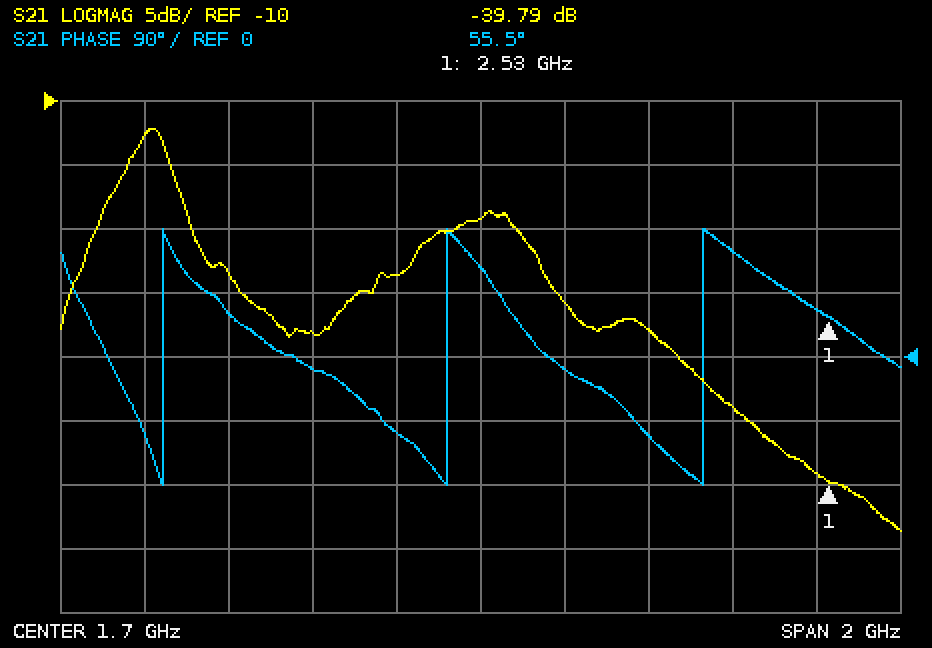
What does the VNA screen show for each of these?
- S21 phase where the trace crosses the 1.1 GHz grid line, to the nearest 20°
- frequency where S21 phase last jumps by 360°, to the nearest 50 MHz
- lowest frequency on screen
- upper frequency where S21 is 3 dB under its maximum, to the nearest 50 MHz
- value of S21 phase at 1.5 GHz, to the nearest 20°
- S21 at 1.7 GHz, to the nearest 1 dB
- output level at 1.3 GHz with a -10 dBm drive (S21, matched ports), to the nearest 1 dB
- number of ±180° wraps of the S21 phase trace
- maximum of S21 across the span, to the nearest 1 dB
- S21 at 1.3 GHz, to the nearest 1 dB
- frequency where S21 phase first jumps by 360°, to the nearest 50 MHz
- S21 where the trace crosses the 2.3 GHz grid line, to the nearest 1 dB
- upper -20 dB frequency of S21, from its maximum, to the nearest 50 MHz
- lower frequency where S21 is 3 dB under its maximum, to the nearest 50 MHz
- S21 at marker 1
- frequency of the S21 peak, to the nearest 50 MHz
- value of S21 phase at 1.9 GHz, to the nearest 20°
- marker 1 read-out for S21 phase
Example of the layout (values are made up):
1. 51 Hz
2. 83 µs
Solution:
1. 60°
2. 2.25 GHz
3. 700 MHz
4. 950 MHz
5. -100°
6. -19 dB
7. -38 dBm
8. 3
9. -12 dB
10. -28 dB
11. 950 MHz
12. -34 dB
13. 2.25 GHz
14. 850 MHz
15. -39.79 dB
16. 900 MHz
17. -20°
18. 55.5°
